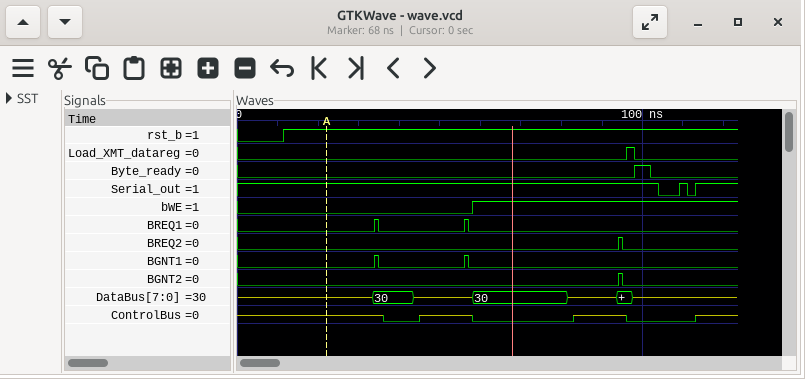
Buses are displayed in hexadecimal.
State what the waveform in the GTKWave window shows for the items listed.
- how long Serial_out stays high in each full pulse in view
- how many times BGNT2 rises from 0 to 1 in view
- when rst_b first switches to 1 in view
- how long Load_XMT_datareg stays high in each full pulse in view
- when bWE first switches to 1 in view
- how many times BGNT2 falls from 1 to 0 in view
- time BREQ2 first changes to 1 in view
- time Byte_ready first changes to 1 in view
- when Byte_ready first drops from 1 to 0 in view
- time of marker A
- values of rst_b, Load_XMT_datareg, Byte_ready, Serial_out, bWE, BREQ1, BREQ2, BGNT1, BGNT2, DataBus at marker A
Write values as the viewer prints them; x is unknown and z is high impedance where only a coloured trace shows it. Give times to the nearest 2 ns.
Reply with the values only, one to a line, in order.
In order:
2 ns
1
12 ns
2 ns
58 ns
1
94 ns
98 ns
102 ns
22 ns
rst_b=1, Load_XMT_datareg=0, Byte_ready=0, Serial_out=1, bWE=0, BREQ1=0, BREQ2=0, BGNT1=0, BGNT2=0, DataBus=z
